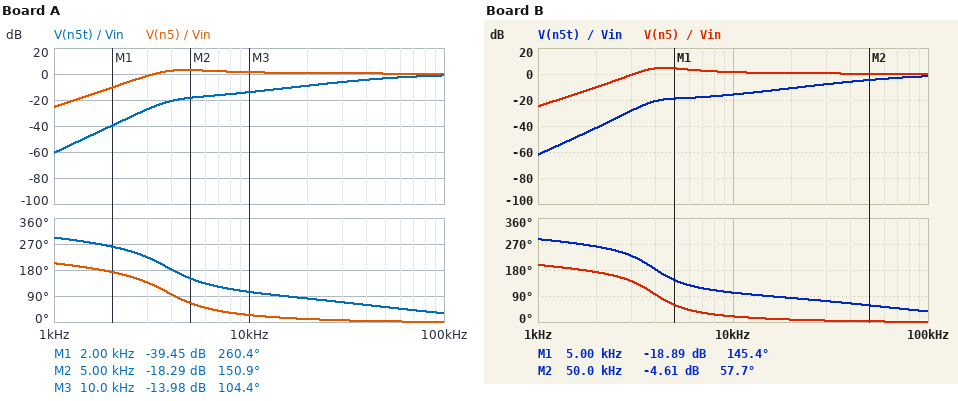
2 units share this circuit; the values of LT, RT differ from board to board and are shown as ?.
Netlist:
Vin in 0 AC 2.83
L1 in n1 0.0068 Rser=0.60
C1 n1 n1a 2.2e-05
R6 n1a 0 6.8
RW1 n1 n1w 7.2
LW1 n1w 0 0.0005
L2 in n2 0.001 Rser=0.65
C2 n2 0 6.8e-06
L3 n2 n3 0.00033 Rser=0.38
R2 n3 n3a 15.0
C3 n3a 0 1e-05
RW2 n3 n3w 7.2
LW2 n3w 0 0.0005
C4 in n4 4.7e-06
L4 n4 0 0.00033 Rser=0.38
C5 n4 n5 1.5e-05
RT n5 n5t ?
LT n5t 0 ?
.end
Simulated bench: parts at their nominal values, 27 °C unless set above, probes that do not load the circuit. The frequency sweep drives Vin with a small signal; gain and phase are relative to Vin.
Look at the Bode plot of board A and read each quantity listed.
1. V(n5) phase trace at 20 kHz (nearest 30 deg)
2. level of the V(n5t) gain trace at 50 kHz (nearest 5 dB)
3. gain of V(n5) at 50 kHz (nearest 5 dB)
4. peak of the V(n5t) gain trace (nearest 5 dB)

0 deg
-5 dB
0 dB
0 dB
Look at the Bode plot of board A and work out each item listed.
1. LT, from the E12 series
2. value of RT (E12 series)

33 µH
12 Ω
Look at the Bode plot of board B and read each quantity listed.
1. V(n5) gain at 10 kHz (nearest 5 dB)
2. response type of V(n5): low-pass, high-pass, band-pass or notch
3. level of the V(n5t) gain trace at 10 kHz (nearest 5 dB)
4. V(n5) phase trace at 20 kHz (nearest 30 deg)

0 dB
high-pass
-15 dB
0 deg
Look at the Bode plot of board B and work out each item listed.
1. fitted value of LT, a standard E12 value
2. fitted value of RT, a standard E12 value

33 µH
15 Ω
